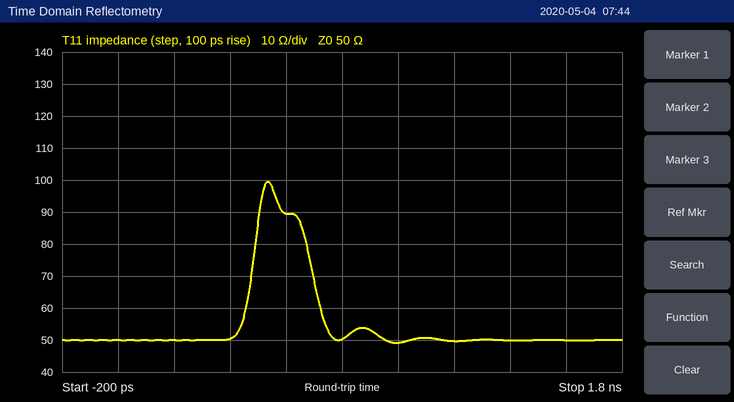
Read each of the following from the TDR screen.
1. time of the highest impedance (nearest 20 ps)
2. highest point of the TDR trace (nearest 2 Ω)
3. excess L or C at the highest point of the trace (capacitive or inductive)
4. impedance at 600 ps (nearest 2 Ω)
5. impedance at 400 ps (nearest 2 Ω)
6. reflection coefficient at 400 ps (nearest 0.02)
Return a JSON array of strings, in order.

["540 ps", "100 Ω", "inductive", "90 Ω", "50 Ω", "0.00"]
